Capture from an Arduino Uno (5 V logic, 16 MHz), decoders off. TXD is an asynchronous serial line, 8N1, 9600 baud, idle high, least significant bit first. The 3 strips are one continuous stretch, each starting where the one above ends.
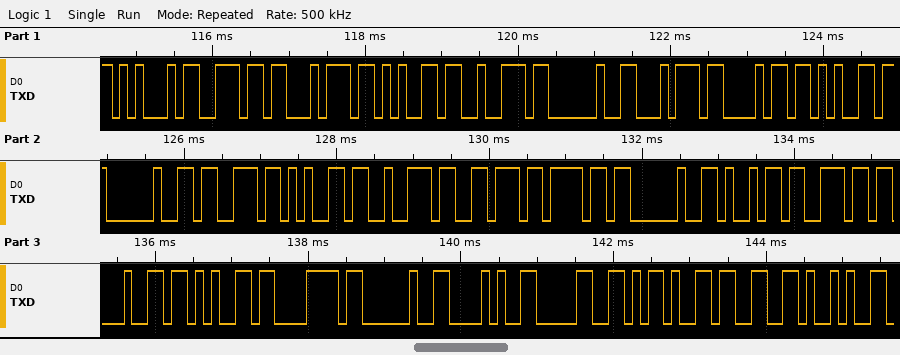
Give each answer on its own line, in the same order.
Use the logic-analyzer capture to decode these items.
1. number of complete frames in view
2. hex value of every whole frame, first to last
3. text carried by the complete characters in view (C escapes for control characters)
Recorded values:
27
45 6E 74 65 72 20 74 68 65 20 73 65 72 76 6F 20 69 6E 64 65 78 20 28 30 2D 33 29
"Enter the servo index (0-3)"
